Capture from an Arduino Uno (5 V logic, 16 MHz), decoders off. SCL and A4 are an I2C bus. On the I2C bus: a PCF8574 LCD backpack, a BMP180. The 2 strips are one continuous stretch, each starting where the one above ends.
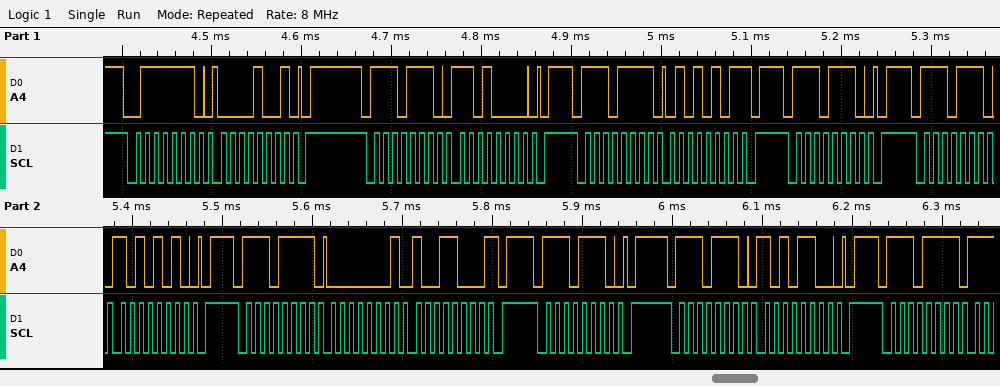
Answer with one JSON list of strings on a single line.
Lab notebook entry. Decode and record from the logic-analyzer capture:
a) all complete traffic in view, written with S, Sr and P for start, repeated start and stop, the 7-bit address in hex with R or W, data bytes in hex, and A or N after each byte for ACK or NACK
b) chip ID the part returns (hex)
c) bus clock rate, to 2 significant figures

["S 3FW A 09 A P S 77W A D0 A P S 77R A 55 N P S 77W A P S 77W A AA A P S 77R A 01 A 98 N P S 77W A P S 77W A AC A P S 77R A", "0x55", "100 kHz"]
